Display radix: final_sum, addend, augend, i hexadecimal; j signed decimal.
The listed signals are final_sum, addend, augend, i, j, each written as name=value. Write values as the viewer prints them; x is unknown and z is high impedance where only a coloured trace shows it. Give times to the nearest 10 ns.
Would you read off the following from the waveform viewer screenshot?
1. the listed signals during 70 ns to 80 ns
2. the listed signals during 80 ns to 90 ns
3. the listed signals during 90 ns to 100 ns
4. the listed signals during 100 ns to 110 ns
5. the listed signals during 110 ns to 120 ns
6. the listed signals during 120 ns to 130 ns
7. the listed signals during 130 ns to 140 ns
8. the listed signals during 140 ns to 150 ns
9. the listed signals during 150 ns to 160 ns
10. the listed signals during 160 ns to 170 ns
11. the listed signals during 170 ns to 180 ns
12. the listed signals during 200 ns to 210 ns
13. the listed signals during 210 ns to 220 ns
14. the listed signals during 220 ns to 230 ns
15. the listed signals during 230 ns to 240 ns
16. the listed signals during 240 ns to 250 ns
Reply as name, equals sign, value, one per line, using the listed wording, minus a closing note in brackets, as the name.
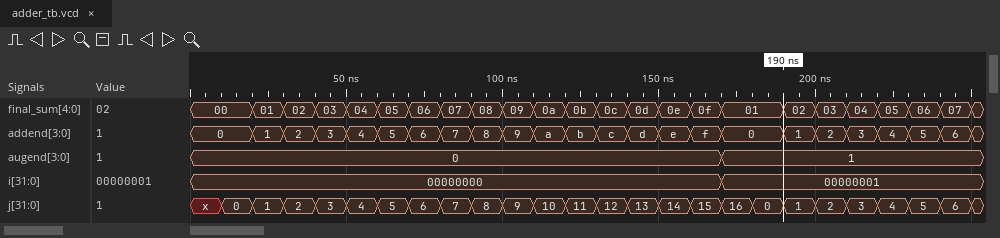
the listed signals during 70 ns to 80 ns = final_sum=06, addend=6, augend=0, i=00000000, j=6
the listed signals during 80 ns to 90 ns = final_sum=07, addend=7, augend=0, i=00000000, j=7
the listed signals during 90 ns to 100 ns = final_sum=08, addend=8, augend=0, i=00000000, j=8
the listed signals during 100 ns to 110 ns = final_sum=09, addend=9, augend=0, i=00000000, j=9
the listed signals during 110 ns to 120 ns = final_sum=0a, addend=a, augend=0, i=00000000, j=10
the listed signals during 120 ns to 130 ns = final_sum=0b, addend=b, augend=0, i=00000000, j=11
the listed signals during 130 ns to 140 ns = final_sum=0c, addend=c, augend=0, i=00000000, j=12
the listed signals during 140 ns to 150 ns = final_sum=0d, addend=d, augend=0, i=00000000, j=13
the listed signals during 150 ns to 160 ns = final_sum=0e, addend=e, augend=0, i=00000000, j=14
the listed signals during 160 ns to 170 ns = final_sum=0f, addend=f, augend=0, i=00000000, j=15
the listed signals during 170 ns to 180 ns = final_sum=01, addend=0, augend=1, i=00000001, j=16
the listed signals during 200 ns to 210 ns = final_sum=03, addend=2, augend=1, i=00000001, j=2
the listed signals during 210 ns to 220 ns = final_sum=04, addend=3, augend=1, i=00000001, j=3
the listed signals during 220 ns to 230 ns = final_sum=05, addend=4, augend=1, i=00000001, j=4
the listed signals during 230 ns to 240 ns = final_sum=06, addend=5, augend=1, i=00000001, j=5
the listed signals during 240 ns to 250 ns = final_sum=07, addend=6, augend=1, i=00000001, j=6
